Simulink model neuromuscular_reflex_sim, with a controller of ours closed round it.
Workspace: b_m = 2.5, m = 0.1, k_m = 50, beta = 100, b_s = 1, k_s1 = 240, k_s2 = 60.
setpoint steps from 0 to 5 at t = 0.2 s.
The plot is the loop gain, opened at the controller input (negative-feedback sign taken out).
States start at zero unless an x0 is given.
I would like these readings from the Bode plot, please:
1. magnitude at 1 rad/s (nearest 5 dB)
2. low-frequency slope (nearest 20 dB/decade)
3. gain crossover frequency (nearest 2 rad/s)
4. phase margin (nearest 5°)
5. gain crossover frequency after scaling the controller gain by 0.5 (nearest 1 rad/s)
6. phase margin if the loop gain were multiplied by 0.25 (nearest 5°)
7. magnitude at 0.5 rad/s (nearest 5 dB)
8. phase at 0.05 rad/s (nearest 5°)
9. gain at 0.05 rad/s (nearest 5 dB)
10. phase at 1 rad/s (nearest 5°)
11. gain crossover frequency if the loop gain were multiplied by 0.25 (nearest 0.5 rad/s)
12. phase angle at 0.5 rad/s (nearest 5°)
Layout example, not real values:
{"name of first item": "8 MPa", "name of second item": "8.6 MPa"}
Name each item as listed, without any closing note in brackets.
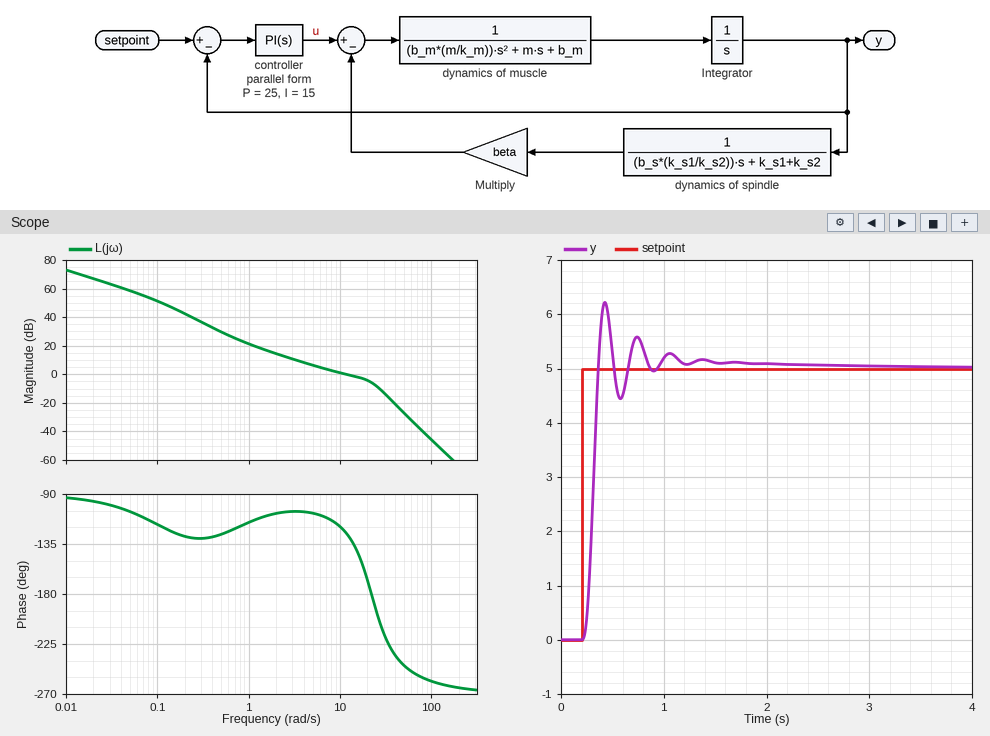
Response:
{"magnitude at 1 rad/s": "20 dB", "low-frequency slope": "-20 dB/decade", "gain crossover frequency": "12 rad/s", "phase margin": "55°", "gain crossover frequency after scaling the controller gain by 0.5": "5 rad/s", "phase margin if the loop gain were multiplied by 0.25": "75°", "magnitude at 0.5 rad/s": "30 dB", "phase at 0.05 rad/s": "-105°", "gain at 0.05 rad/s": "60 dB", "phase at 1 rad/s": "-115°", "gain crossover frequency if the loop gain were multiplied by 0.25": "2.5 rad/s", "phase angle at 0.5 rad/s": "-125°"}
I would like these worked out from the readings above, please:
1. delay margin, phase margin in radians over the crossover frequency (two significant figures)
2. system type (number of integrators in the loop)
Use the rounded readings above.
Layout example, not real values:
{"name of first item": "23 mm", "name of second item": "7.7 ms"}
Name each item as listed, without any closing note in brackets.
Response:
{"delay margin, phase margin in radians over the crossover frequency": "0.080 s", "system type": "1"}
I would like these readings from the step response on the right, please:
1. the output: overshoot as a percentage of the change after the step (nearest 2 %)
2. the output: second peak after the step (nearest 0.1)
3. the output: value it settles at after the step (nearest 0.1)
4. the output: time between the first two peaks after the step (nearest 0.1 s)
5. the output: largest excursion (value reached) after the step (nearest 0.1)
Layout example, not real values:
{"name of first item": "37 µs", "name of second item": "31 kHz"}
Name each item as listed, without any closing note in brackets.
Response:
{"the output: overshoot as a percentage of the change after the step": "24 %", "the output: second peak after the step": "5.6", "the output: value it settles at after the step": "5.0", "the output: time between the first two peaks after the step": "0.3 s", "the output: largest excursion (value reached) after the step": "6.2"}
